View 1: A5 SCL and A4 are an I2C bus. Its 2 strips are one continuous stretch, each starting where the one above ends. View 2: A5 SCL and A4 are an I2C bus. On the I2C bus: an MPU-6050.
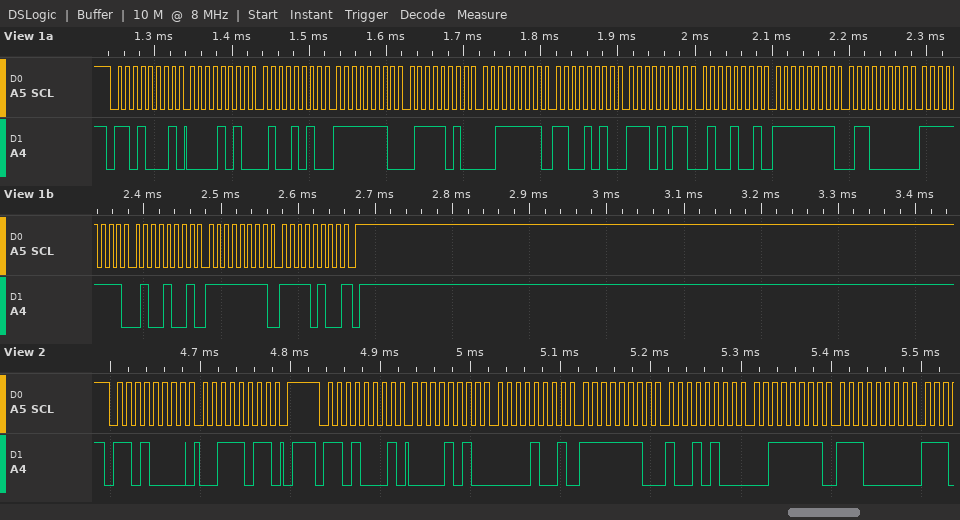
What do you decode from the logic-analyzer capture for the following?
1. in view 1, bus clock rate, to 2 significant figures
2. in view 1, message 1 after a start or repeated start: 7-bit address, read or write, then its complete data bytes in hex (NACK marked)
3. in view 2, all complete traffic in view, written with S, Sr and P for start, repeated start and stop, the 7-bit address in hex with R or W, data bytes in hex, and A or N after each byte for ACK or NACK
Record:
100 kHz
0x68 read: 0A 4A FE 7A 3F CA EB 49 FF 60 FF 49 FF F4 NACK
S 68W A 3B A P S 68R A 0A A 09 A FE A 94 A 3F A E0 A
